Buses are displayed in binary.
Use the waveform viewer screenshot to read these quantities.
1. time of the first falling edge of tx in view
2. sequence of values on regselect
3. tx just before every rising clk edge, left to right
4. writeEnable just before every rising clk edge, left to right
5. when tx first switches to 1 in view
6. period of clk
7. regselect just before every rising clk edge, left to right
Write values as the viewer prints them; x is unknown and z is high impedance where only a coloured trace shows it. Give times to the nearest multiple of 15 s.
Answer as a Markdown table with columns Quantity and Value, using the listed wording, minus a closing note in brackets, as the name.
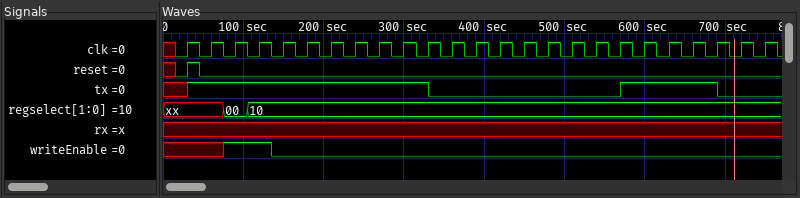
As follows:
| Quantity | Value |
|---|---|
| time of the first falling edge of tx in view | 330 s |
| sequence of values on regselect | xx, 00, 10 |
| tx just before every rising clk edge, left to right | x 1 1 1 1 1 1 1 1 1 1 0 0 0 0 0 0 0 0 1 1 1 1 0 0 |
| writeEnable just before every rising clk edge, left to right | x x 1 1 0 0 0 0 0 0 0 0 0 0 0 0 0 0 0 0 0 0 0 0 0 |
| when tx first switches to 1 in view | 30 s |
| period of clk | 30 s |
| regselect just before every rising clk edge, left to right | xx, xx, 00, 10, 10, 10, 10, 10, 10, 10, 10, 10, 10, 10, 10, 10, 10, 10, 10, 10, 10, 10, 10, 10, 10 |
